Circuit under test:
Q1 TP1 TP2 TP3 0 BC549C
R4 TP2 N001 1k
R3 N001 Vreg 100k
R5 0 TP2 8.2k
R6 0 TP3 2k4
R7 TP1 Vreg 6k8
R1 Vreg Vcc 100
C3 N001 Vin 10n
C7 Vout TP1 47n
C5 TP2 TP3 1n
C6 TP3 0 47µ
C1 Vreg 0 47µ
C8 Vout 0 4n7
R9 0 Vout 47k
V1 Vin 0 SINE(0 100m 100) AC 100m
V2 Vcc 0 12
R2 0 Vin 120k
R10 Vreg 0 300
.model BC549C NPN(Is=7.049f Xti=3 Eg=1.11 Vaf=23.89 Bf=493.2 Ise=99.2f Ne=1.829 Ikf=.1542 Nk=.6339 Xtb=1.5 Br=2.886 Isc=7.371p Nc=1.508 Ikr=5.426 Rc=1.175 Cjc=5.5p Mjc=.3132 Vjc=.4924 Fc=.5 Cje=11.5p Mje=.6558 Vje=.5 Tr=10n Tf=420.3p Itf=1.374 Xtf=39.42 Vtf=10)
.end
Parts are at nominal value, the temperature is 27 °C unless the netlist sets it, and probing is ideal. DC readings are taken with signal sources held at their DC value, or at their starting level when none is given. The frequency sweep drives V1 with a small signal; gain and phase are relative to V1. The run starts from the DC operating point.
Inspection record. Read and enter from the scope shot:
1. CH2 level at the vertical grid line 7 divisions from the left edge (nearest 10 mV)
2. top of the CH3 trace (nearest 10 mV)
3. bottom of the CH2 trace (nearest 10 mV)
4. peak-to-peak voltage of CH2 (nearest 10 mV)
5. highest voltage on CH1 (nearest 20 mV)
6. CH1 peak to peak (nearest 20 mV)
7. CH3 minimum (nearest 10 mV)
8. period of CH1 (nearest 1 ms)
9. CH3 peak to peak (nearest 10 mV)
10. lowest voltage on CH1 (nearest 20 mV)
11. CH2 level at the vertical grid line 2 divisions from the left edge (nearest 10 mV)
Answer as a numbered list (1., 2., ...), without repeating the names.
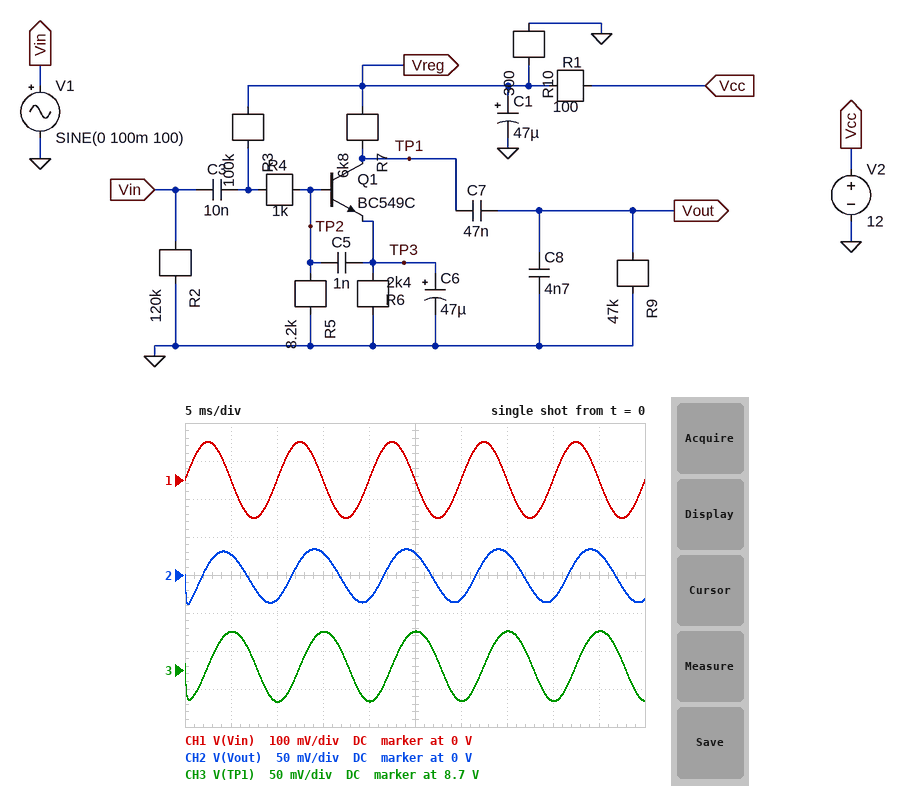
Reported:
1. 30 mV
2. 8.75 V
3. -40 mV
4. 70 mV
5. 100 mV
6. 200 mV
7. 8.66 V
8. 10 ms
9. 90 mV
10. -100 mV
11. -30 mV
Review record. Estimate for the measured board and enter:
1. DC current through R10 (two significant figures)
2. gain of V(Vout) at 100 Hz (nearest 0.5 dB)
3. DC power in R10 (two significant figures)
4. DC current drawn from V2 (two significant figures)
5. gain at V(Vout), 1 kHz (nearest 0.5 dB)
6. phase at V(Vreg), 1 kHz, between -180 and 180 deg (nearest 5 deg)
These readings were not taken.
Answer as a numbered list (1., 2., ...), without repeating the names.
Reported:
1. 30 mA
2. -9.0 dB
3. 270 mW
4. 30 mA
5. 11.0 dB
6. 145 deg
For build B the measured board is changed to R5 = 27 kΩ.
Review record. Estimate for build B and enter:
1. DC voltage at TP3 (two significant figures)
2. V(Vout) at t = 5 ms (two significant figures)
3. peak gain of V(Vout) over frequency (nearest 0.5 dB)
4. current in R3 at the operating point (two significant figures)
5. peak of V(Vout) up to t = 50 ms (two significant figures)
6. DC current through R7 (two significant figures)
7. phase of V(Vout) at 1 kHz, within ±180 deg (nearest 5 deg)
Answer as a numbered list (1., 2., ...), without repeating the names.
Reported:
1. 1.2 V
2. 360 mV
3. 37.0 dB
4. 70 µA
5. 550 mV
6. 510 µA
7. -135 deg
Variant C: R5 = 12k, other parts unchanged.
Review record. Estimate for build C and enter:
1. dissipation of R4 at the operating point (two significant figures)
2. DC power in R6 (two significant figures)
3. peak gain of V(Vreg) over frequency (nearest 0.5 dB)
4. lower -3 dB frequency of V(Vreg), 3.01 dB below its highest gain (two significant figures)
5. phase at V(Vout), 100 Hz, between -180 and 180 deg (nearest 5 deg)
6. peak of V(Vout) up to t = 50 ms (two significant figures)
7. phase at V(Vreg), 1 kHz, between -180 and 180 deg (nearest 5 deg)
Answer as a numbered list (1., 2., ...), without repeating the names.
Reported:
1. 6.3 µW
2. 49 µW
3. -40.5 dB
4. 45 Hz
5. -55 deg
6. 150 mV
7. 140 deg
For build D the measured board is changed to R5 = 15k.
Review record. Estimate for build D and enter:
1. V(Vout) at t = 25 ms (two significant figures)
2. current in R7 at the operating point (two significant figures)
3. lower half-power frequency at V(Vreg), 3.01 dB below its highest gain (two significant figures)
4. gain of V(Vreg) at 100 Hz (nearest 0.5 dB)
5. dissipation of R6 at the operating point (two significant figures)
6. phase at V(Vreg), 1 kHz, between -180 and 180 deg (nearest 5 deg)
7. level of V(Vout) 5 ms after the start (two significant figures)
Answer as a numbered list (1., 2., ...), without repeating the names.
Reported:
1. 190 mV
2. 220 µA
3. 50 Hz
4. -36.5 dB
5. 120 µW
6. 135 deg
7. 170 mV
